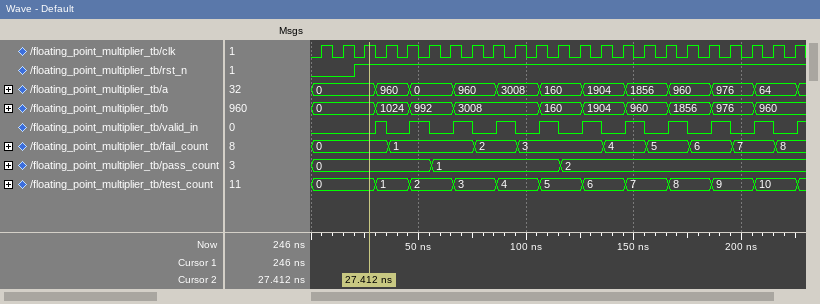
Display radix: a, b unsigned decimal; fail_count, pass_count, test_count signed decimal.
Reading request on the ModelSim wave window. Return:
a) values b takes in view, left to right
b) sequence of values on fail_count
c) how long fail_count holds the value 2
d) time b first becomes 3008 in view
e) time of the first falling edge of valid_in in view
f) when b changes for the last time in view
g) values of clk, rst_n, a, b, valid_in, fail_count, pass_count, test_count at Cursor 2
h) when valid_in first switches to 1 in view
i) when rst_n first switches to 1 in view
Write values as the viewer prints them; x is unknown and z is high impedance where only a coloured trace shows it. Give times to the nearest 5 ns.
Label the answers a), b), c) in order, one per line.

a) 0, 1024, 992, 3008, 160, 1904, 960, 1856, 976, 960
b) 0, 1, 2, 3, 4, 5, 6, 7, 8
c) 20 ns
d) 65 ns
e) 35 ns
f) 205 ns
g) clk=1, rst_n=1, a=0, b=0, valid_in=0, fail_count=0, pass_count=0, test_count=0
h) 30 ns
i) 20 ns
